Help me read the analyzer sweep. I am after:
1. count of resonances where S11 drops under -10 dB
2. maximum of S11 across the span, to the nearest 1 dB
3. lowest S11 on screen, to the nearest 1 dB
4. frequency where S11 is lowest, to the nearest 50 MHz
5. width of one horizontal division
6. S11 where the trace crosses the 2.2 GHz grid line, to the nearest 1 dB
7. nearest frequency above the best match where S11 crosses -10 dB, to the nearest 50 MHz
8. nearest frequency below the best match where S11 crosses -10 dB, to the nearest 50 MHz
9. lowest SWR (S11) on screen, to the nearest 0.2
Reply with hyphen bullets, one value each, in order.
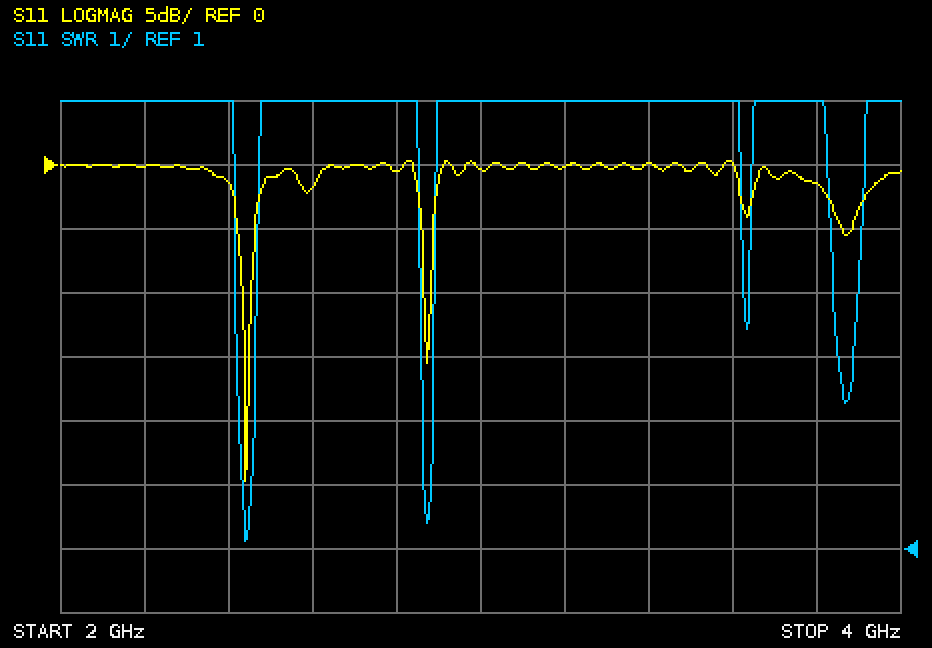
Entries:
- 2
- 0 dB
- -25 dB
- 2.45 GHz
- 200 MHz
- 0 dB
- 2.45 GHz
- 2.45 GHz
- 1.2
